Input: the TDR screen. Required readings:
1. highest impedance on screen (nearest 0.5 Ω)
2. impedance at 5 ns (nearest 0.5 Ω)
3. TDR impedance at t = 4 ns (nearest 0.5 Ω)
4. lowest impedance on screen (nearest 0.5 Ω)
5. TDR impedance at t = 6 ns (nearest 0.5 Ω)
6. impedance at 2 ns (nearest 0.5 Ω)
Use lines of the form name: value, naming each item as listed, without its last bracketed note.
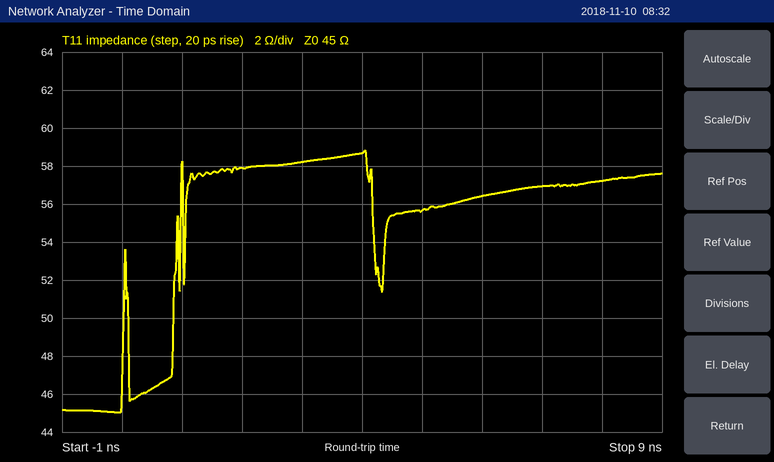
highest impedance on screen: 59.0 Ω
impedance at 5 ns: 55.5 Ω
TDR impedance at t = 4 ns: 58.5 Ω
lowest impedance on screen: 45.0 Ω
TDR impedance at t = 6 ns: 56.5 Ω
impedance at 2 ns: 58.0 Ω
